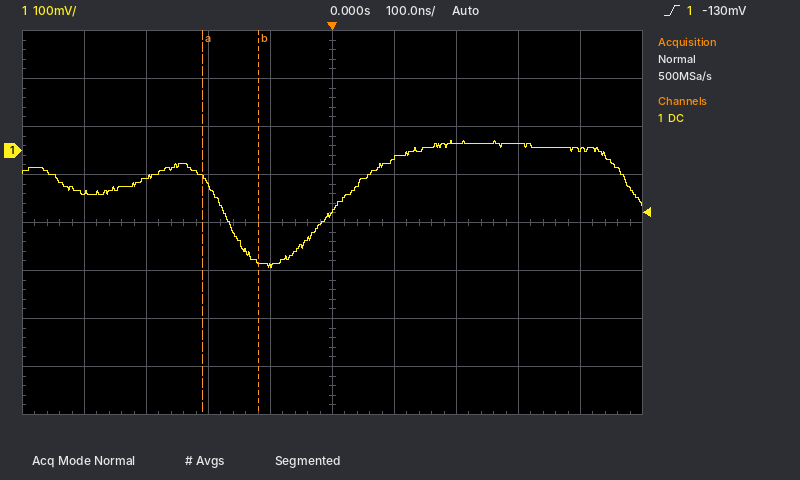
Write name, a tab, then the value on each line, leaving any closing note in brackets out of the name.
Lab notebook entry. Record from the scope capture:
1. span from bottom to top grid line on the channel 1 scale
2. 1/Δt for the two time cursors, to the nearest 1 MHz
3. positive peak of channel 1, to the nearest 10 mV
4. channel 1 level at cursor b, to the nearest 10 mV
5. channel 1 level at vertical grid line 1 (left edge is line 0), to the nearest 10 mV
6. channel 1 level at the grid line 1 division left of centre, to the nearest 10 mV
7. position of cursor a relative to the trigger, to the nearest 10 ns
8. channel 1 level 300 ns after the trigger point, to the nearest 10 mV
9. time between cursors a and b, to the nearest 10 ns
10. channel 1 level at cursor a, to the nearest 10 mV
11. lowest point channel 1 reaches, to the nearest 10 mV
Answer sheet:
span from bottom to top grid line on the channel 1 scale	800 mV
1/Δt for the two time cursors, to the nearest 1 MHz	11 MHz
positive peak of channel 1, to the nearest 10 mV	20 mV
channel 1 level at cursor b, to the nearest 10 mV	-230 mV
channel 1 level at vertical grid line 1 (left edge is line 0), to the nearest 10 mV	-90 mV
channel 1 level at the grid line 1 division left of centre, to the nearest 10 mV	-240 mV
position of cursor a relative to the trigger, to the nearest 10 ns	-210 ns
channel 1 level 300 ns after the trigger point, to the nearest 10 mV	10 mV
time between cursors a and b, to the nearest 10 ns	90 ns
channel 1 level at cursor a, to the nearest 10 mV	-60 mV
lowest point channel 1 reaches, to the nearest 10 mV	-240 mV
